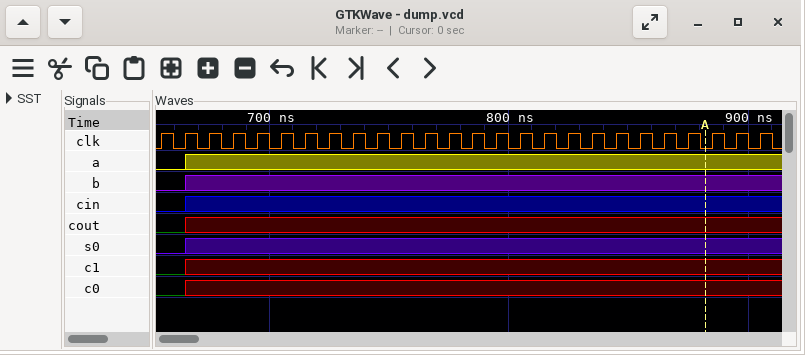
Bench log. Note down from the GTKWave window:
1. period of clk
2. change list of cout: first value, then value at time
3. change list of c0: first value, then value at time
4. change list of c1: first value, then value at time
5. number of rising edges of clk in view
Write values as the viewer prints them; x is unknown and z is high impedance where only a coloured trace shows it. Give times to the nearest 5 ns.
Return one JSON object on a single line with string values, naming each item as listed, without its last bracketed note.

{"period of clk": "10 ns", "change list of cout: first value, then value at time": "0, x at 665 ns", "change list of c0: first value, then value at time": "0, x at 665 ns", "change list of c1: first value, then value at time": "0, x at 665 ns", "number of rising edges of clk in view": "26"}
